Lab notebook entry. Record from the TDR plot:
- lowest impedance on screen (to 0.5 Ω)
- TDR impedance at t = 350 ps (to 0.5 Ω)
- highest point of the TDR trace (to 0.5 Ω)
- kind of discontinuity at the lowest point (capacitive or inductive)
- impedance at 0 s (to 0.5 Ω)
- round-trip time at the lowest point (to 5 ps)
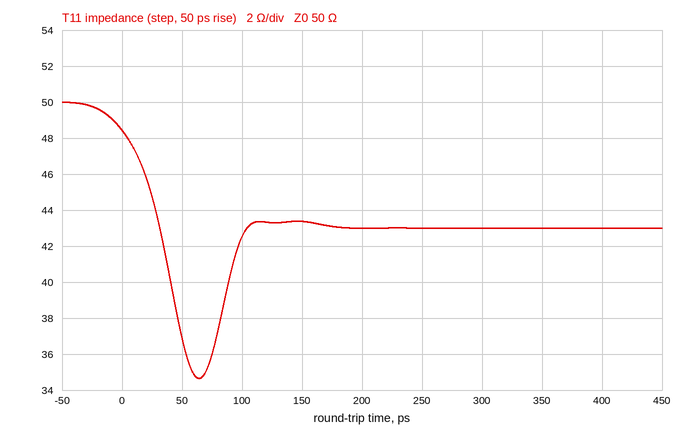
34.5 Ω
43.0 Ω
50.0 Ω
capacitive
48.5 Ω
65 ps
